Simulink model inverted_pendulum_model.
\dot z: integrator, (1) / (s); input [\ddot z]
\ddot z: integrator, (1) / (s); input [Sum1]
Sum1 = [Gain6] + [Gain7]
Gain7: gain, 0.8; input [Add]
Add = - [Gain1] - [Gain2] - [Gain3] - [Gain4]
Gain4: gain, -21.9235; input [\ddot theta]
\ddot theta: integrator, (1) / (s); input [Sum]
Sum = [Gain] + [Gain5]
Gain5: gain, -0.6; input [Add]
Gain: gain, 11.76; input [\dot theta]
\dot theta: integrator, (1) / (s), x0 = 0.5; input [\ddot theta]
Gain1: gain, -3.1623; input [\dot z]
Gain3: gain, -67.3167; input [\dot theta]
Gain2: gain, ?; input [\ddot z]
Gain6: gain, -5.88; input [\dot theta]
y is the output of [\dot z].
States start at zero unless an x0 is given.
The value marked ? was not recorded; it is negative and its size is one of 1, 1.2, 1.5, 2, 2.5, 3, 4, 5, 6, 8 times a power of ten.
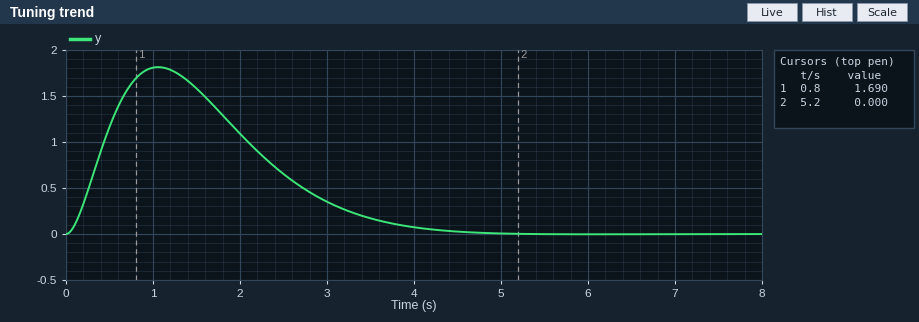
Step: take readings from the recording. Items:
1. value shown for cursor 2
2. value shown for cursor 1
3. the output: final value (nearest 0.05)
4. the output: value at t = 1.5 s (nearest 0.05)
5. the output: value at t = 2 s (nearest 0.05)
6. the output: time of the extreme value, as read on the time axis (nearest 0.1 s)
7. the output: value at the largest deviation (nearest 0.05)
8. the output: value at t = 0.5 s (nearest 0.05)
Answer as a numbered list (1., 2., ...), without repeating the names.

1. 0.000
2. 1.690
3. 0.00
4. 1.60
5. 1.10
6. 1.1 s
7. 1.80
8. 1.15
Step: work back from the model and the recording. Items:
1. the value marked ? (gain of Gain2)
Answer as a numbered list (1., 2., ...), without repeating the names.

1. -6
